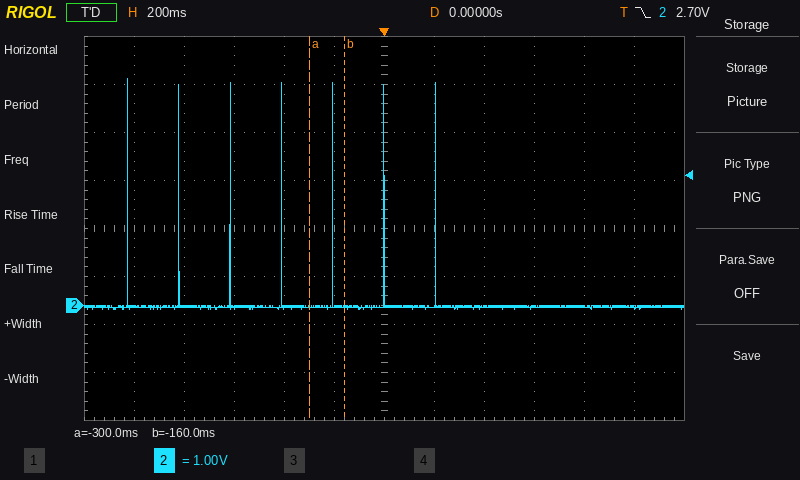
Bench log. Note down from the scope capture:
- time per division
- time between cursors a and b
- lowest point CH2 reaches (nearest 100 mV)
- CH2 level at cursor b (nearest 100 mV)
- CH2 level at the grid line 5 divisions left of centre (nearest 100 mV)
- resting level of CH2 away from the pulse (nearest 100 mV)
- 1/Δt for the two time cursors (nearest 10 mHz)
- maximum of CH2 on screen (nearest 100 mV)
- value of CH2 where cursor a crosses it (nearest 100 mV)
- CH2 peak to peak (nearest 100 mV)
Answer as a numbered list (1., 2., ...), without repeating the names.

1. 200 ms
2. 140 ms
3. -100 mV
4. 0.0 V
5. 0.0 V
6. 0.0 V
7. 7.14 Hz
8. 4.7 V
9. 0.0 V
10. 4.8 V
